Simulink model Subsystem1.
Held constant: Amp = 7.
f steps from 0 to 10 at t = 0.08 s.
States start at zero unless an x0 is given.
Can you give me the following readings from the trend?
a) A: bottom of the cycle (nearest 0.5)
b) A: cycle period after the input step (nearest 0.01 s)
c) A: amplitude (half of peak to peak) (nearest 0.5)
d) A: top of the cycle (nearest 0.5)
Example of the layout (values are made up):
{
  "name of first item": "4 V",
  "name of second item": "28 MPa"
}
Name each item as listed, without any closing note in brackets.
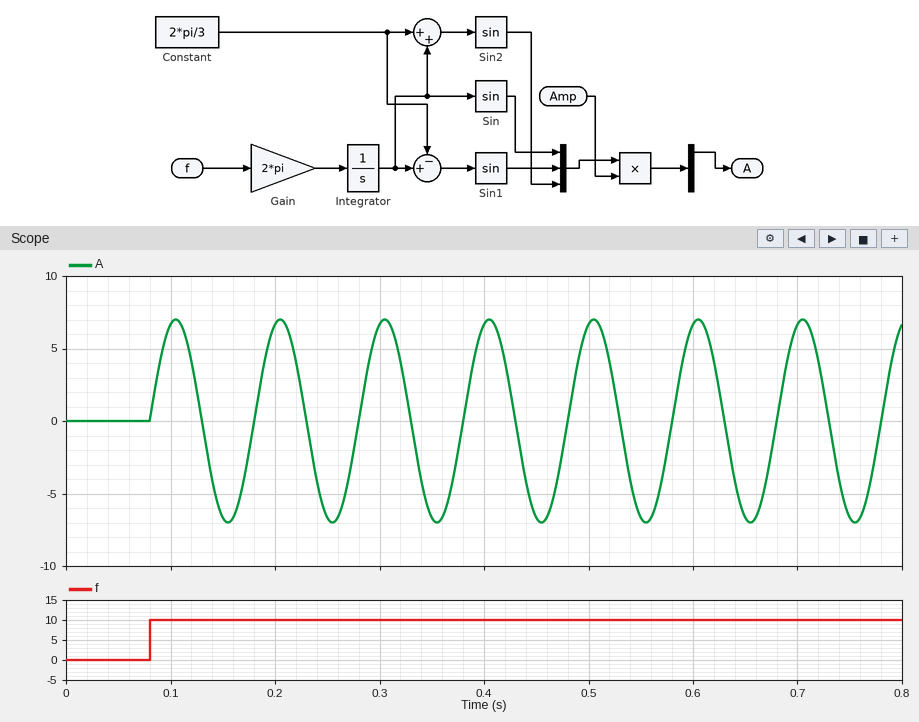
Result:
{
  "A: bottom of the cycle": "-7.0",
  "A: cycle period after the input step": "0.10 s",
  "A: amplitude (half of peak to peak)": "7.0",
  "A: top of the cycle": "7.0"
}
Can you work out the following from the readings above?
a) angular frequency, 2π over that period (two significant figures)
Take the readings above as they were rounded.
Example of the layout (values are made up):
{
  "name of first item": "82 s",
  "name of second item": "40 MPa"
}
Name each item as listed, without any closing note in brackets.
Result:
{
  "angular frequency, 2π over that period": "63 rad/s"
}
